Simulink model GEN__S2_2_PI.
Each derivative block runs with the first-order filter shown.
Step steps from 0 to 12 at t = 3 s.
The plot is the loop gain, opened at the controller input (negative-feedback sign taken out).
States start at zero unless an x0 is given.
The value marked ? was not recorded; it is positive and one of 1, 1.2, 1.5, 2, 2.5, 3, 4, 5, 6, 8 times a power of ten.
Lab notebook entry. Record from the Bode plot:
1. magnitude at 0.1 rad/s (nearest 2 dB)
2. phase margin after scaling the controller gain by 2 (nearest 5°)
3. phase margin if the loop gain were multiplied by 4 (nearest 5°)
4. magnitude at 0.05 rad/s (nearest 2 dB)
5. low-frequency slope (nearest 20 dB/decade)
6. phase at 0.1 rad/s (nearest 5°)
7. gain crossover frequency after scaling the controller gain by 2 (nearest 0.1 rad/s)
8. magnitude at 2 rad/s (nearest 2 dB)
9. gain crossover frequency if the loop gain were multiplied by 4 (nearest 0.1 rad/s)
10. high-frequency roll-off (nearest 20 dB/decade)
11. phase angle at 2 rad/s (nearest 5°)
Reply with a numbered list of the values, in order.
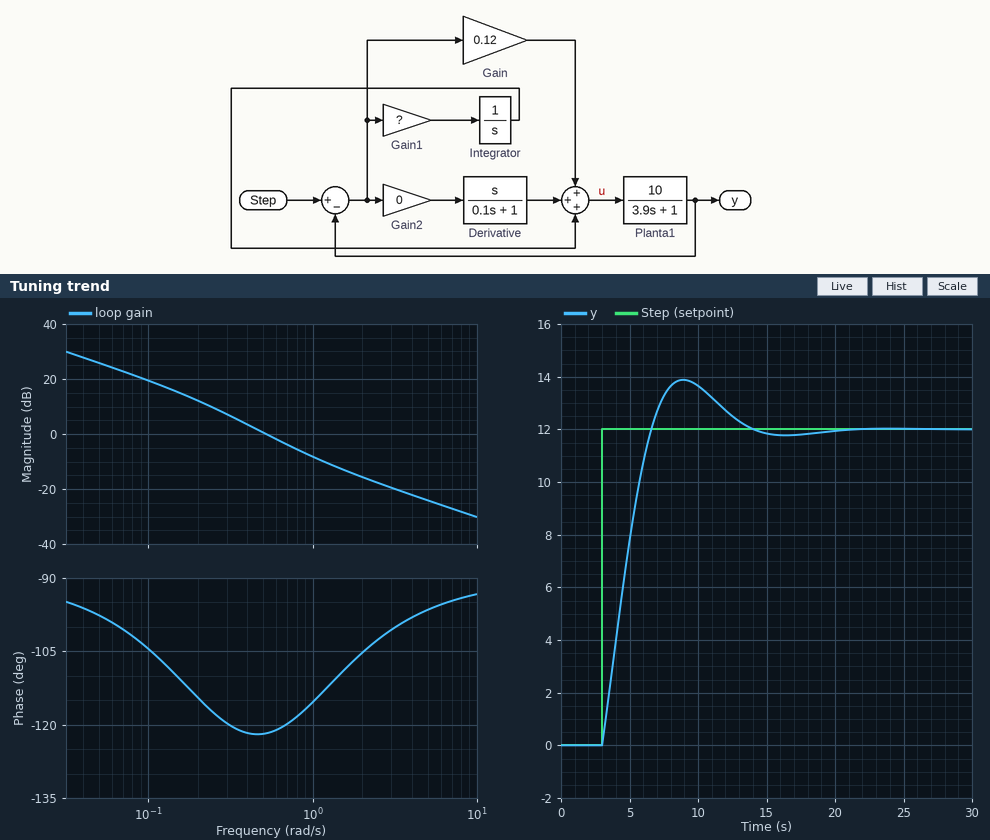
1. 20 dB
2. 60°
3. 70°
4. 26 dB
5. -20 dB/decade
6. -105°
7. 0.8 rad/s
8. -16 dB
9. 1.4 rad/s
10. -20 dB/decade
11. -105°
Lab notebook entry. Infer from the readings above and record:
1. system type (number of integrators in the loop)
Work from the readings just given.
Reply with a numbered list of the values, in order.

1. 1
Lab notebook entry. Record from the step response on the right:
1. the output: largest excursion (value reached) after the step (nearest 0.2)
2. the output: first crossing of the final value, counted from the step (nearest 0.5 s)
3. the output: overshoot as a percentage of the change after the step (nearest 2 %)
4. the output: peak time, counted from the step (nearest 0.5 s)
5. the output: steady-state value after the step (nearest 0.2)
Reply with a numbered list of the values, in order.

1. 13.8
2. 3.5 s
3. 16 %
4. 6.0 s
5. 12.0
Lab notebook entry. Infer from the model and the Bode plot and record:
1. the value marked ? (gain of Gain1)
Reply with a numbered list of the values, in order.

1. 0.1
